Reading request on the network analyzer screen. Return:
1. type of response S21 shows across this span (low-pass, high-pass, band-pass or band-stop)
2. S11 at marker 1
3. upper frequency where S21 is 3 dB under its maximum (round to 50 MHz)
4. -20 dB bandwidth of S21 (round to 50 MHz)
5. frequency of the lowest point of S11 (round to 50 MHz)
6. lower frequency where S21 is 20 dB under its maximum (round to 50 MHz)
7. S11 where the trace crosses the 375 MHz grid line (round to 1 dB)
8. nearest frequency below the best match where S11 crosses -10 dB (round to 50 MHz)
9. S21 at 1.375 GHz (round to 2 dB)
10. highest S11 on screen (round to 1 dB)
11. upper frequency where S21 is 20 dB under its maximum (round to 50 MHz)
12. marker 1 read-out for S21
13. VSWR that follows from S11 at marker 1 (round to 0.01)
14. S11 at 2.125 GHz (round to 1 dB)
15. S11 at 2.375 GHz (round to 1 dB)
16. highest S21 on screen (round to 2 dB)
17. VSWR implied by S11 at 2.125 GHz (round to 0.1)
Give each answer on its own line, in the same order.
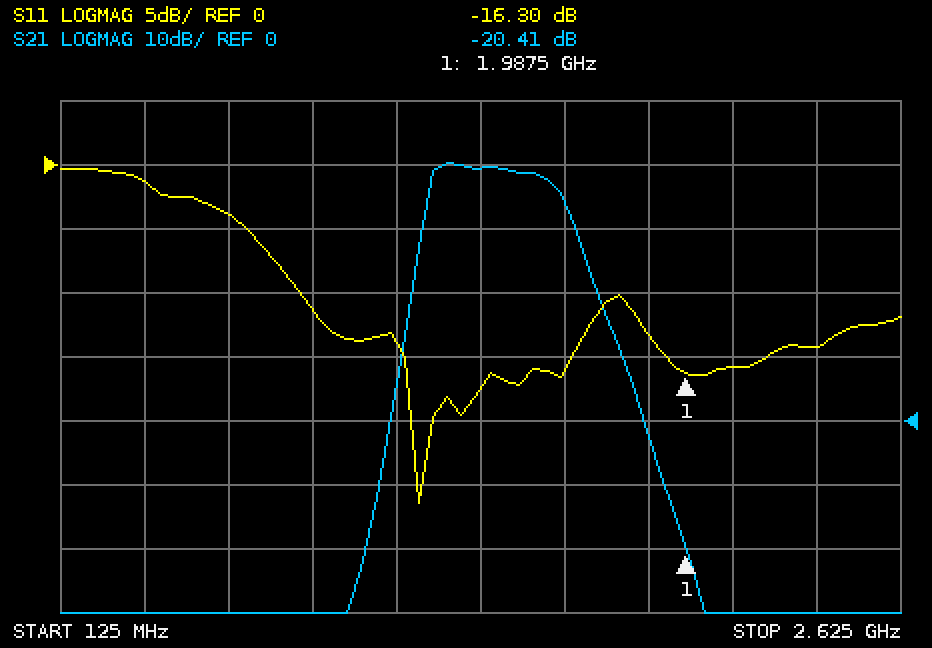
band-pass
-16.30 dB
1.60 GHz
550 MHz
1.20 GHz
1.15 GHz
-1 dB
850 MHz
40 dB
0 dB
1.70 GHz
-20.41 dB
1.36
-16 dB
-14 dB
40 dB
1.4
